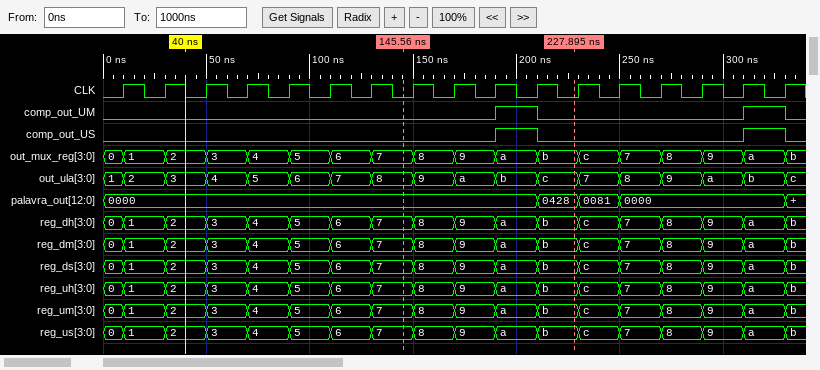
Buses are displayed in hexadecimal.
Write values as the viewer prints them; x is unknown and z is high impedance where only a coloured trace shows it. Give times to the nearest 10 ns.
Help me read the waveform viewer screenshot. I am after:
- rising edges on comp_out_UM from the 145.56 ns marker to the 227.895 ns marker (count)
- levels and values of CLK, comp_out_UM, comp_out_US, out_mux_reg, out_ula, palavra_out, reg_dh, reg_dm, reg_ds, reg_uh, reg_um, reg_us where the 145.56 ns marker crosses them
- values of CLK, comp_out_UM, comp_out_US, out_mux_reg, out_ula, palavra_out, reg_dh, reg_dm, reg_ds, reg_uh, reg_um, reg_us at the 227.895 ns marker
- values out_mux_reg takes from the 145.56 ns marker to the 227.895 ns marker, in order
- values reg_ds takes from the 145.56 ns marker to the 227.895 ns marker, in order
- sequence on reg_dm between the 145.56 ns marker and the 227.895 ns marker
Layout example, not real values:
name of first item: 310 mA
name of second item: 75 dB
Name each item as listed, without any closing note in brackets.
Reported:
rising edges on comp_out_UM from the 145.56 ns marker to the 227.895 ns marker: 1
levels and values of CLK, comp_out_UM, comp_out_US, out_mux_reg, out_ula, palavra_out, reg_dh, reg_dm, reg_ds, reg_uh, reg_um, reg_us where the 145.56 ns marker crosses them: CLK=0, comp_out_UM=0, comp_out_US=0, out_mux_reg=7, out_ula=8, palavra_out=0000, reg_dh=7, reg_dm=7, reg_ds=7, reg_uh=7, reg_um=7, reg_us=7
values of CLK, comp_out_UM, comp_out_US, out_mux_reg, out_ula, palavra_out, reg_dh, reg_dm, reg_ds, reg_uh, reg_um, reg_us at the 227.895 ns marker: CLK=0, comp_out_UM=0, comp_out_US=0, out_mux_reg=b, out_ula=c, palavra_out=0428, reg_dh=b, reg_dm=b, reg_ds=b, reg_uh=b, reg_um=b, reg_us=b
values out_mux_reg takes from the 145.56 ns marker to the 227.895 ns marker, in order: 7, 8, 9, a, b
values reg_ds takes from the 145.56 ns marker to the 227.895 ns marker, in order: 7, 8, 9, a, b
sequence on reg_dm between the 145.56 ns marker and the 227.895 ns marker: 7, 8, 9, a, b
